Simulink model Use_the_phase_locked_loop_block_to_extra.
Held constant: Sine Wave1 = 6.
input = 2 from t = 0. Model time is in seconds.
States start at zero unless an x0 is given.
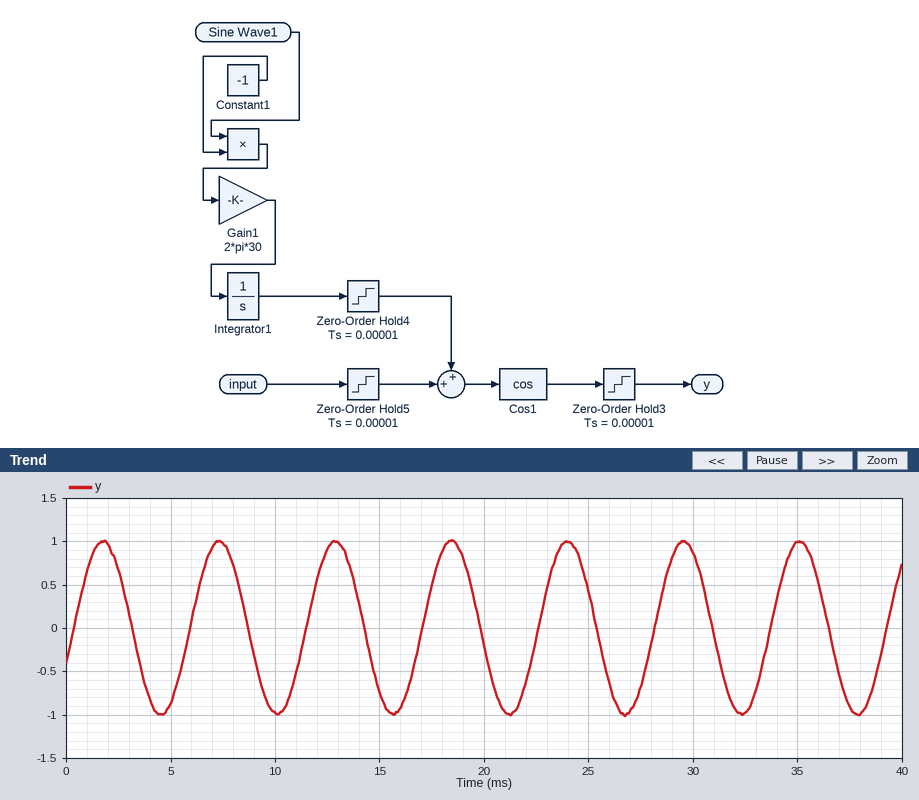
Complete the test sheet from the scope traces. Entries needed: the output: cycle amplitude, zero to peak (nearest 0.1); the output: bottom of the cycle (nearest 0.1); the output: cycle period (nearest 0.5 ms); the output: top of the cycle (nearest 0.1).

1.0
-1.0
5.5 ms
1.0
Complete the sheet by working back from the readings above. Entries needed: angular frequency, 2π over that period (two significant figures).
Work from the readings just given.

1.1 rad/ms
